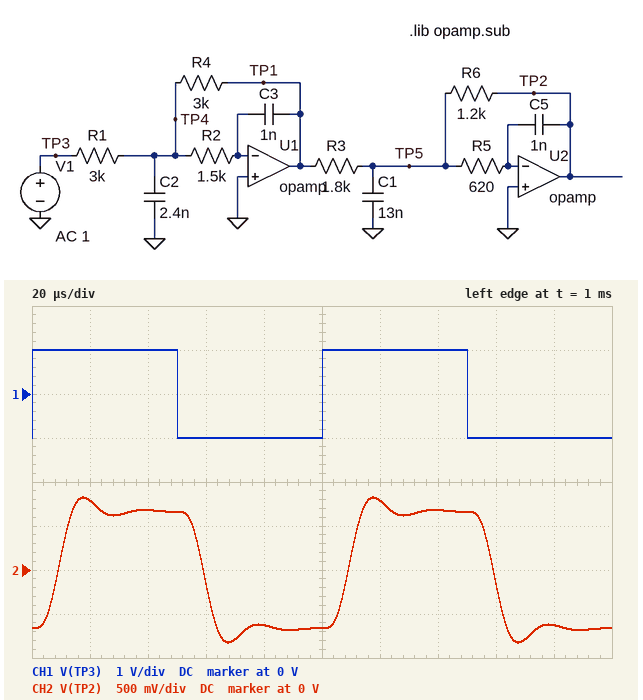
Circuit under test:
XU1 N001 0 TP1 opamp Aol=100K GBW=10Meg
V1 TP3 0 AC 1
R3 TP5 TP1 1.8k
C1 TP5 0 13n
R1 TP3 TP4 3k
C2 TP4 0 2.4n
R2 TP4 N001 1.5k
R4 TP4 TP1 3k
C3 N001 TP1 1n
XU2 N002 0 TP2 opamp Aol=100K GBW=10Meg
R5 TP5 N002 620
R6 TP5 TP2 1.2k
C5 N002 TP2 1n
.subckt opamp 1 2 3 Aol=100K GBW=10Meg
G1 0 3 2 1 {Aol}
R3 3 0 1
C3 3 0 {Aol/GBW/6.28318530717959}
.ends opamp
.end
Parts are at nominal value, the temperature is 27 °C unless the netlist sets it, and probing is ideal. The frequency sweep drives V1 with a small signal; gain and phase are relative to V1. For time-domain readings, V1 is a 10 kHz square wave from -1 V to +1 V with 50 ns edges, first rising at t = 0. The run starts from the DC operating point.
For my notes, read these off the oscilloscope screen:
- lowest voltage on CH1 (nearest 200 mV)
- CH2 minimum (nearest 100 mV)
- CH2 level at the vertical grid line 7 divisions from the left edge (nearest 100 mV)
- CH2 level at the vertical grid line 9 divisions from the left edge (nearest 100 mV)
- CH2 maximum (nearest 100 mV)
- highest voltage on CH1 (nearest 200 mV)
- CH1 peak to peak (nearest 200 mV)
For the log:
-1.0 V
-800 mV
700 mV
-600 mV
800 mV
1.0 V
2.0 V
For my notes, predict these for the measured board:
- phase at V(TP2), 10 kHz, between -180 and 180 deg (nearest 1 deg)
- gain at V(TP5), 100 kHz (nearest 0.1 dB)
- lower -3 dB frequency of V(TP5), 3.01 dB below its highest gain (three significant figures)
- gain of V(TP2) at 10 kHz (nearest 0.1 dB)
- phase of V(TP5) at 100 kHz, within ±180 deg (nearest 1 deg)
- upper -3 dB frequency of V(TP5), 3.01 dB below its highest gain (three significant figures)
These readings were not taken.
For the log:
-30 deg
-35.7 dB
27.8 kHz
-3.5 dB
-16 deg
59.4 kHz
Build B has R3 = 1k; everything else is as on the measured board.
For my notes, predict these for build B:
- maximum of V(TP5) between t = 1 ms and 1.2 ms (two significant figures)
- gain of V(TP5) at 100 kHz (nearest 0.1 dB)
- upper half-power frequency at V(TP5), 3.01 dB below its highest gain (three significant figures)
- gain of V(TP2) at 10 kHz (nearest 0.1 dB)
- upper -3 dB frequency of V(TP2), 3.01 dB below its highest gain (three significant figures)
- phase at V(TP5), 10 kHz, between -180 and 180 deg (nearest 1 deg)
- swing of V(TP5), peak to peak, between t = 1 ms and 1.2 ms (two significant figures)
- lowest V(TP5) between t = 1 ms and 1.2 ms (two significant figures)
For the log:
180 mV
-30.9 dB
59.5 kHz
1.6 dB
47.8 kHz
-121 deg
350 mV
-180 mV
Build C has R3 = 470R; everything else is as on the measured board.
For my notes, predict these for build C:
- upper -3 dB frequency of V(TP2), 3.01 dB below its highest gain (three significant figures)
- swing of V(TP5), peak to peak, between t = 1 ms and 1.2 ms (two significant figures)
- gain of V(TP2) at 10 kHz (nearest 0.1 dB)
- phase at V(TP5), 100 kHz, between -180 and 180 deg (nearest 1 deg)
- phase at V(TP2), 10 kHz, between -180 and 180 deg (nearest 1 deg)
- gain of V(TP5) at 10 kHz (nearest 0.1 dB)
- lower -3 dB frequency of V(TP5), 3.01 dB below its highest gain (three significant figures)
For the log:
38.9 kHz
660 mV
8.0 dB
-5 deg
-34 deg
-19.9 dB
20.8 kHz
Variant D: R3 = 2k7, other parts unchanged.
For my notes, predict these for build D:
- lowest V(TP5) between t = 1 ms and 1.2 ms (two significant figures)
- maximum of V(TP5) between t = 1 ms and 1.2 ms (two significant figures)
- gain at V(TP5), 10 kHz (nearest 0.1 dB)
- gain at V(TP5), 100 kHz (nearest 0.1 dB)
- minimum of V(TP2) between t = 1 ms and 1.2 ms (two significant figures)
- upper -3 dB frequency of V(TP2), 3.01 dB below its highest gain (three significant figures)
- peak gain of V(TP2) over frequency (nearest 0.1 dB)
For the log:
-71 mV
71 mV
-35.0 dB
-39.1 dB
-560 mV
52.3 kHz
-6.8 dB
